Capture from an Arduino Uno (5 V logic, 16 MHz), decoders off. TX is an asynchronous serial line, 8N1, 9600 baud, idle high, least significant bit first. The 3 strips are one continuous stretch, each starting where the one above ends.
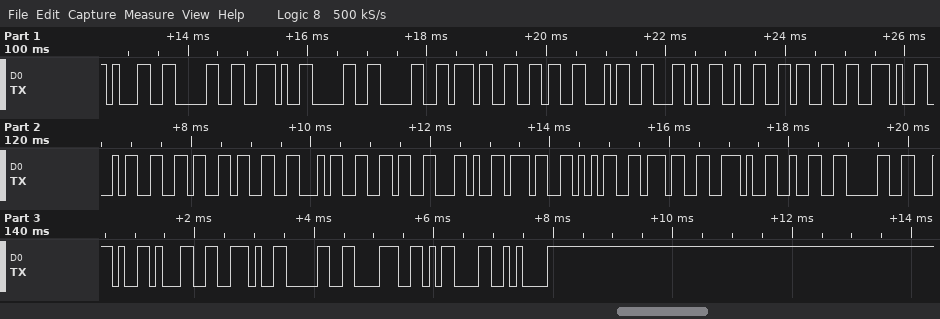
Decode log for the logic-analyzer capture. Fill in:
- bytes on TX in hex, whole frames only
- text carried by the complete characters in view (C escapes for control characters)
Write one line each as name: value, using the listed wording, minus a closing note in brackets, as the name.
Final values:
bytes on TX in hex, whole frames only: 31 30 2E 30 30 37 36 34 2C 32 33 2E 34 36 33 34 36 2C 37 35 37 2E 32 30 2C 31 2E 30 38 0D 0A
text carried by the complete characters in view: "10.00764,23.46346,757.20,1.08\r\n"
